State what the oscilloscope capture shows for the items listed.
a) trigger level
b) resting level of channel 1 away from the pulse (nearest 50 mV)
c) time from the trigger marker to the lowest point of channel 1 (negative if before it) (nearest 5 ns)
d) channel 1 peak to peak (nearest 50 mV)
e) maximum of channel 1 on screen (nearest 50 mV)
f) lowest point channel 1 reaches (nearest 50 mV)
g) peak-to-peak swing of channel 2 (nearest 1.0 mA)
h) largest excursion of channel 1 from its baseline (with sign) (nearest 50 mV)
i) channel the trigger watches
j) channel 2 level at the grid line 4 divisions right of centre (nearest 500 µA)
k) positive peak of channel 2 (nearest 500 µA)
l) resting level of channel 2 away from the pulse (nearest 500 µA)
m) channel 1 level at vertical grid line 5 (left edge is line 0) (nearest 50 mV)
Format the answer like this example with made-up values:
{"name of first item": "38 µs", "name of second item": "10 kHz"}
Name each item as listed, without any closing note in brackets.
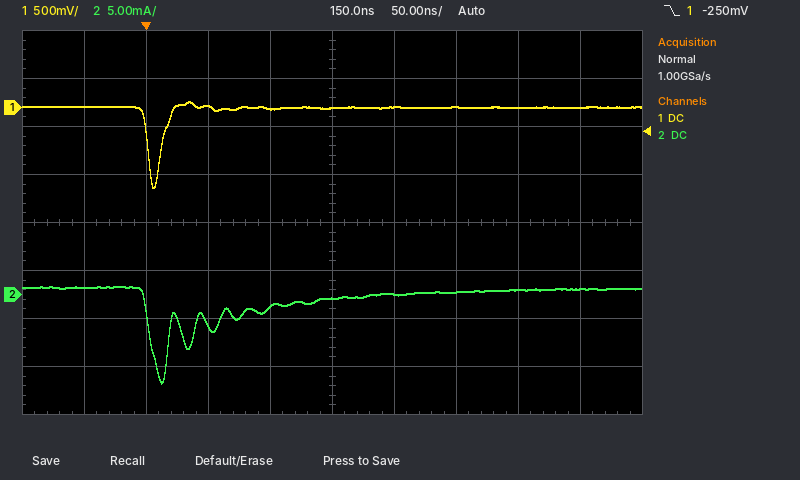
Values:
{"trigger level": "-250 mV", "resting level of channel 1 away from the pulse": "0 mV", "time from the trigger marker to the lowest point of channel 1 (negative if before it)": "+5 ns", "channel 1 peak to peak": "900 mV", "maximum of channel 1 on screen": "50 mV", "lowest point channel 1 reaches": "-850 mV", "peak-to-peak swing of channel 2": "10.0 mA", "largest excursion of channel 1 from its baseline (with sign)": "-850 mV", "channel the trigger watches": "channel 1", "channel 2 level at the grid line 4 divisions right of centre": "500 µA", "positive peak of channel 2": "1.0 mA", "resting level of channel 2 away from the pulse": "500 µA", "channel 1 level at vertical grid line 5 (left edge is line 0)": "0 mV"}
